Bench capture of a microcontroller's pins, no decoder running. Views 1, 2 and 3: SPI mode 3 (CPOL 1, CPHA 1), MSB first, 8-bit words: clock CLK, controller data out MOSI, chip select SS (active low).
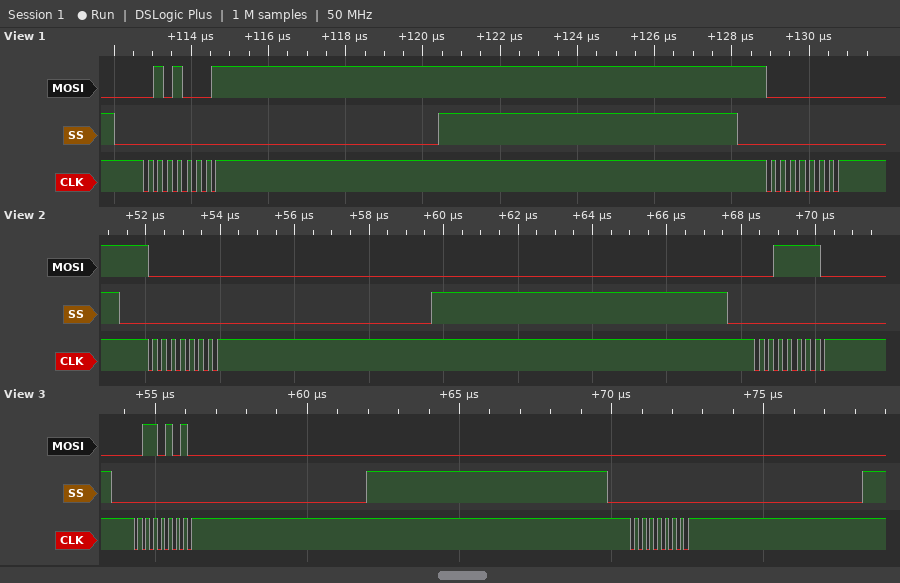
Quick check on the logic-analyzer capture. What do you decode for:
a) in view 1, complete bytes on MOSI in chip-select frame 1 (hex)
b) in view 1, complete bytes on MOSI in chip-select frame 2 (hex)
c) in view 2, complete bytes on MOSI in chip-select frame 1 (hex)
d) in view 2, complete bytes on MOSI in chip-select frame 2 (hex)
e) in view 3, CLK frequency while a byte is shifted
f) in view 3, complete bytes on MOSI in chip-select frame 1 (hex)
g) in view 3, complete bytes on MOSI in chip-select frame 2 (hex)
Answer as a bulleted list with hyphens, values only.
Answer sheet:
- 51
- 00
- 00
- 3E
- 4 MHz
- 6A
- 00
